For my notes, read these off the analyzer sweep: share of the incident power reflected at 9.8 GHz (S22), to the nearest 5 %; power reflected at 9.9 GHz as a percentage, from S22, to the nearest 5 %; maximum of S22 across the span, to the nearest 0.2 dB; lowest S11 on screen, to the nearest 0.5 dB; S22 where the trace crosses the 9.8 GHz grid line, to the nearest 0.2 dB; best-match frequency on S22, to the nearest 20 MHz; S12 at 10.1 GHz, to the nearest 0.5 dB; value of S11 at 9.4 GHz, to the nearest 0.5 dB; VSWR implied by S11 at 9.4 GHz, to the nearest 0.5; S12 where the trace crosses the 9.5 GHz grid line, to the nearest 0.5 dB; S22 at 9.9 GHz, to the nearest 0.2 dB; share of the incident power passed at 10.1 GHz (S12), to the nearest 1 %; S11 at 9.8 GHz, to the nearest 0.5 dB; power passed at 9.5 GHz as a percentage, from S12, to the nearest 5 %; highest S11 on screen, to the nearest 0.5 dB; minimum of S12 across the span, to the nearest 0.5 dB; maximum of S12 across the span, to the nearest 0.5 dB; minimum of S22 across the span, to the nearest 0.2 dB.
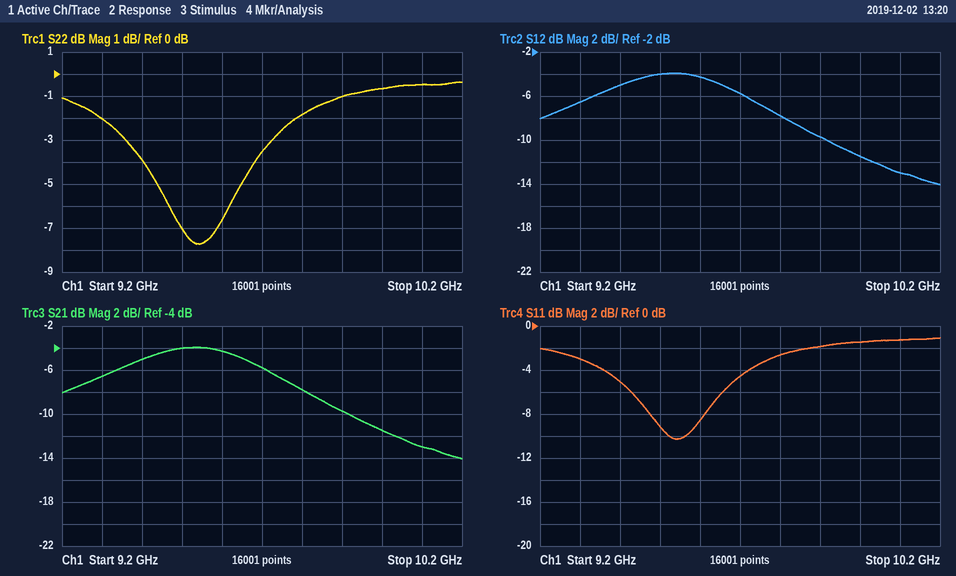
65 %
80 %
-0.4 dB
-10.5 dB
-1.8 dB
9.54 GHz
-13.0 dB
-5.0 dB
3.5
-4.0 dB
-1.0 dB
5 %
-2.5 dB
40 %
-1.0 dB
-14.0 dB
-4.0 dB
-7.8 dB
